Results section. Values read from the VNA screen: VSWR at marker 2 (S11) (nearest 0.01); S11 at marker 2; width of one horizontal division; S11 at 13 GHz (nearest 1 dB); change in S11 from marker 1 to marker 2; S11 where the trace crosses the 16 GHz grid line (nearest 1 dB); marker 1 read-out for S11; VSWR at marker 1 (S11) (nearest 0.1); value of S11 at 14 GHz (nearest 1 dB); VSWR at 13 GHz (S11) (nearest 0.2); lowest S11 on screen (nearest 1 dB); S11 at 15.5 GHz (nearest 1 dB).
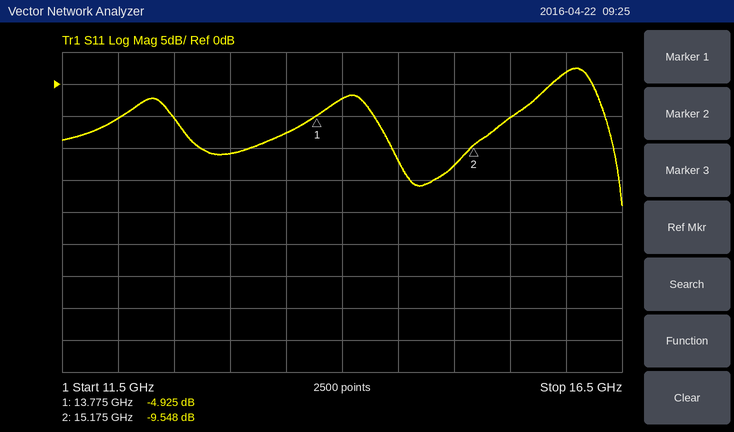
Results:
2.00
-9.548 dB
500 MHz
-11 dB
-4.623 dB
2 dB
-4.925 dB
3.6
-2 dB
1.8
-19 dB
-5 dB
